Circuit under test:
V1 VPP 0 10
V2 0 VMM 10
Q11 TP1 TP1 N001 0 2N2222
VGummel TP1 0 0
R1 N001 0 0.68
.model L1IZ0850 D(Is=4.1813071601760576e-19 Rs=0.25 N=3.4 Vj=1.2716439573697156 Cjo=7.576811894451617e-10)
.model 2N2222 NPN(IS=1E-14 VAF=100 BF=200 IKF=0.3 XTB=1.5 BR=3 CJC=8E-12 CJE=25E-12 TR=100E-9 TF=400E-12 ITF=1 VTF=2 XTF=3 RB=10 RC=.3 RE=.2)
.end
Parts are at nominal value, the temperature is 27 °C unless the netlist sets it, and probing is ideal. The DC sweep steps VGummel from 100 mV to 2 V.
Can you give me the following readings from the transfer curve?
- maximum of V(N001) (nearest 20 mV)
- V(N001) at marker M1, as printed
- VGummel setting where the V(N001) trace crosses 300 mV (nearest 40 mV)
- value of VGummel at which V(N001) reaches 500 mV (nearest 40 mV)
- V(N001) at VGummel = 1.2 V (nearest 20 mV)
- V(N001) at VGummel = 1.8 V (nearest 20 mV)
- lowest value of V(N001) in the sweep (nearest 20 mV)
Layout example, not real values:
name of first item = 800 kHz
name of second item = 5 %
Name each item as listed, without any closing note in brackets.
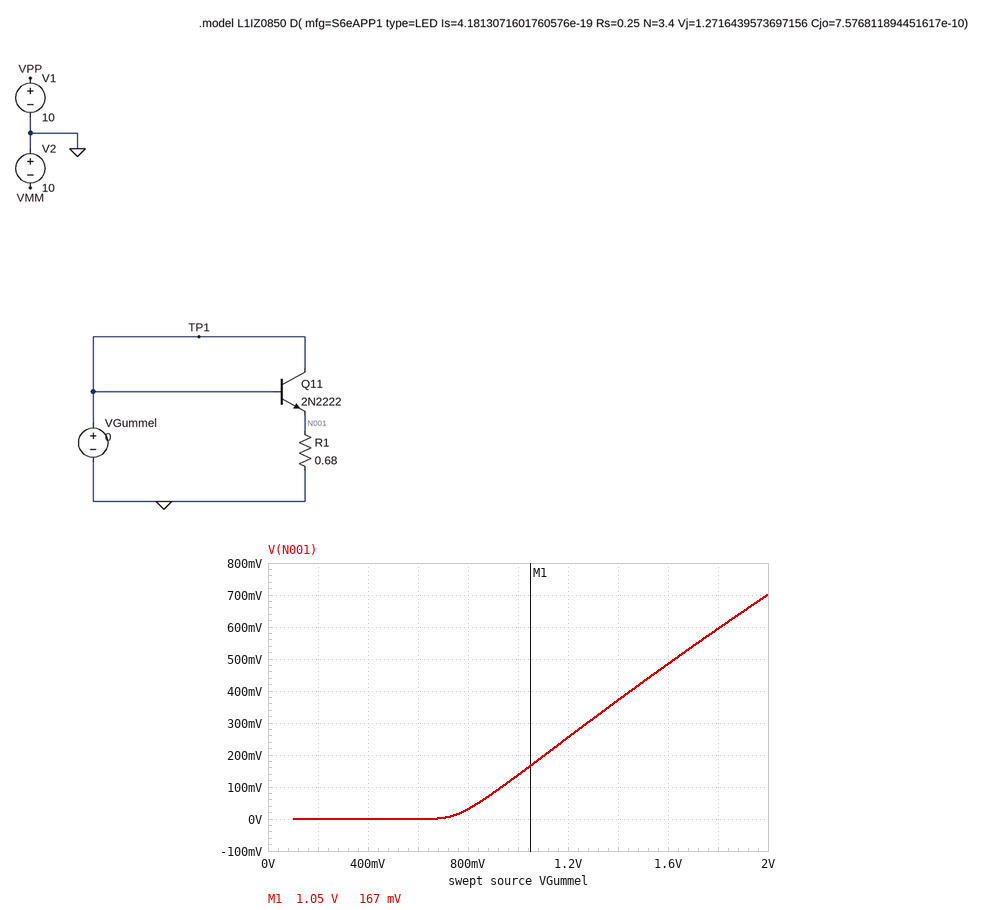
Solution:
maximum of V(N001) = 700 mV
V(N001) at marker M1, as printed = 167 mV
VGummel setting where the V(N001) trace crosses 300 mV = 1.28 V
value of VGummel at which V(N001) reaches 500 mV = 1.64 V
V(N001) at VGummel = 1.2 V = 260 mV
V(N001) at VGummel = 1.8 V = 600 mV
lowest value of V(N001) in the sweep = 0 V
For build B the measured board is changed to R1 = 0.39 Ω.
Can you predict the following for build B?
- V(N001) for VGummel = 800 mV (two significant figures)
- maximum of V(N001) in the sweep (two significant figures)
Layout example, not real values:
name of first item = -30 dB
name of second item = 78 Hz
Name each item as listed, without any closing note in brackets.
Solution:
V(N001) for VGummel = 800 mV = 22 mV
maximum of V(N001) in the sweep = 510 mV
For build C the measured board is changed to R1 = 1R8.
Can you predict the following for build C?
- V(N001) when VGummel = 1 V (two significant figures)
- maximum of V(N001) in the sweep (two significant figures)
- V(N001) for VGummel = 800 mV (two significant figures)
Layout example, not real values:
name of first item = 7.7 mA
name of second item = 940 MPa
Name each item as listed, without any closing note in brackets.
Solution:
V(N001) when VGummel = 1 V = 190 mV
maximum of V(N001) in the sweep = 970 mV
V(N001) for VGummel = 800 mV = 50 mV
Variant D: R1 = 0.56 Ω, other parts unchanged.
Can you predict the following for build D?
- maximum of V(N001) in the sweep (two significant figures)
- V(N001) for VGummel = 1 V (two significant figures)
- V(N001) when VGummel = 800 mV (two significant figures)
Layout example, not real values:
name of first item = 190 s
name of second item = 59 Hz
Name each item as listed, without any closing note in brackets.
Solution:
maximum of V(N001) in the sweep = 640 mV
V(N001) for VGummel = 1 V = 130 mV
V(N001) when VGummel = 800 mV = 28 mV
